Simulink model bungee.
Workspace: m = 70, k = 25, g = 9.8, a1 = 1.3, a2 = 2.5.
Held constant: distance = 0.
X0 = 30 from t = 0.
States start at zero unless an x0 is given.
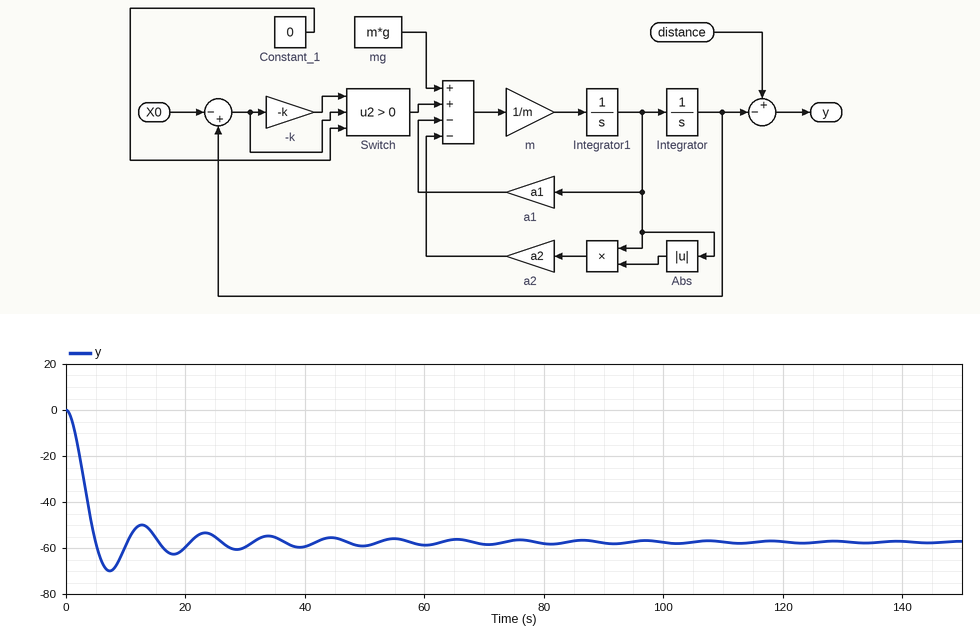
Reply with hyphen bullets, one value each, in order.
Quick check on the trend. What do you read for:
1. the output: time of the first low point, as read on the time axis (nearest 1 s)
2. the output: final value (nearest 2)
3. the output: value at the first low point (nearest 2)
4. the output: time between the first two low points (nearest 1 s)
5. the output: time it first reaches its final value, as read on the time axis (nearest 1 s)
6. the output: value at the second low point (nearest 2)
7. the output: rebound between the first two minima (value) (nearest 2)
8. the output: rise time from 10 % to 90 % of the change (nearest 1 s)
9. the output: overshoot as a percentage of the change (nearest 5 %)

- 7 s
- -58
- -70
- 11 s
- 5 s
- -62
- -50
- 3 s
- 20 %
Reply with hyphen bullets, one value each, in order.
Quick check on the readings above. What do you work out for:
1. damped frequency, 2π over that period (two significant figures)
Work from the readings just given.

- 0.57 rad/s
